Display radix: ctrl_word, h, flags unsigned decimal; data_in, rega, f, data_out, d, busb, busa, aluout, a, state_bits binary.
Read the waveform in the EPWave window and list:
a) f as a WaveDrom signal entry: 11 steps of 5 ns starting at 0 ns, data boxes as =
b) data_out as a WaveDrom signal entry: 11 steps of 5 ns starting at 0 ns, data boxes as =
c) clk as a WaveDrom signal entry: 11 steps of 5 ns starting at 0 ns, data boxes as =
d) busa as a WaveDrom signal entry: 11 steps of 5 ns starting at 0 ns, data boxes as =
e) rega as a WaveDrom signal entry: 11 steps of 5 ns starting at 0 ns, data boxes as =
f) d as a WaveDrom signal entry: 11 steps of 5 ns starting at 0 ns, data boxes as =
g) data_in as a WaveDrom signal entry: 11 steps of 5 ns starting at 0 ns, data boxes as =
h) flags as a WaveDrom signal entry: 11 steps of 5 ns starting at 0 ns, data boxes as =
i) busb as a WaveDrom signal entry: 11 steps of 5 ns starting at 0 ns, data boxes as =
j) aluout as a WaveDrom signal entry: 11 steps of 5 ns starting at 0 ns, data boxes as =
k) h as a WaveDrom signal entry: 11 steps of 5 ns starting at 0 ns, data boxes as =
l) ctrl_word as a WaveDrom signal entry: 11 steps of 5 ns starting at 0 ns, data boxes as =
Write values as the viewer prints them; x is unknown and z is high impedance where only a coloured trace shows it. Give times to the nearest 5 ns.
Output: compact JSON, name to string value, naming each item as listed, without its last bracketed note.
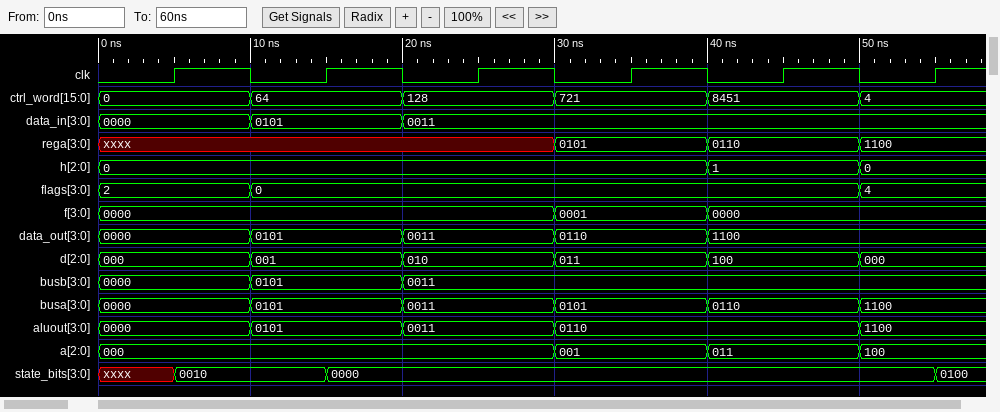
{"f as a WaveDrom signal entry: 11 steps of 5 ns starting at 0 ns, data boxes as =": "{name: 'f', wave: '=.....=.=..', data: '0000 0001 0000'}", "data_out as a WaveDrom signal entry: 11 steps of 5 ns starting at 0 ns, data boxes as =": "{name: 'data_out', wave: '=.=.=.=.=..', data: '0000 0101 0011 0110 1100'}", "clk as a WaveDrom signal entry: 11 steps of 5 ns starting at 0 ns, data boxes as =": "{name: 'clk', wave: '01010101010'}", "busa as a WaveDrom signal entry: 11 steps of 5 ns starting at 0 ns, data boxes as =": "{name: 'busa', wave: '=.=.=.=.=.=', data: '0000 0101 0011 0101 0110 1100'}", "rega as a WaveDrom signal entry: 11 steps of 5 ns starting at 0 ns, data boxes as =": "{name: 'rega', wave: 'x.....=.=.=', data: '0101 0110 1100'}", "d as a WaveDrom signal entry: 11 steps of 5 ns starting at 0 ns, data boxes as =": "{name: 'd', wave: '=.=.=.=.=.=', data: '000 001 010 011 100 000'}", "data_in as a WaveDrom signal entry: 11 steps of 5 ns starting at 0 ns, data boxes as =": "{name: 'data_in', wave: '=.=.=......', data: '0000 0101 0011'}", "flags as a WaveDrom signal entry: 11 steps of 5 ns starting at 0 ns, data boxes as =": "{name: 'flags', wave: '=.=.......=', data: '2 0 4'}", "busb as a WaveDrom signal entry: 11 steps of 5 ns starting at 0 ns, data boxes as =": "{name: 'busb', wave: '=.=.=......', data: '0000 0101 0011'}", "aluout as a WaveDrom signal entry: 11 steps of 5 ns starting at 0 ns, data boxes as =": "{name: 'aluout', wave: '=.=.=.=...=', data: '0000 0101 0011 0110 1100'}", "h as a WaveDrom signal entry: 11 steps of 5 ns starting at 0 ns, data boxes as =": "{name: 'h', wave: '=.......=.=', data: '0 1 0'}", "ctrl_word as a WaveDrom signal entry: 11 steps of 5 ns starting at 0 ns, data boxes as =": "{name: 'ctrl_word', wave: '=.=.=.=.=.=', data: '0 64 128 721 8451 4'}"}
